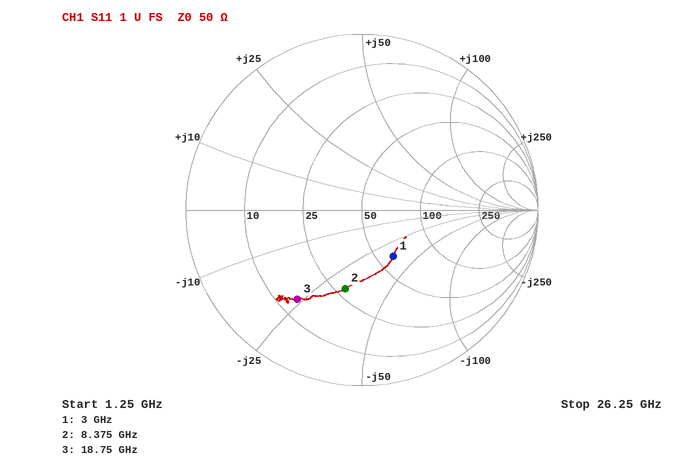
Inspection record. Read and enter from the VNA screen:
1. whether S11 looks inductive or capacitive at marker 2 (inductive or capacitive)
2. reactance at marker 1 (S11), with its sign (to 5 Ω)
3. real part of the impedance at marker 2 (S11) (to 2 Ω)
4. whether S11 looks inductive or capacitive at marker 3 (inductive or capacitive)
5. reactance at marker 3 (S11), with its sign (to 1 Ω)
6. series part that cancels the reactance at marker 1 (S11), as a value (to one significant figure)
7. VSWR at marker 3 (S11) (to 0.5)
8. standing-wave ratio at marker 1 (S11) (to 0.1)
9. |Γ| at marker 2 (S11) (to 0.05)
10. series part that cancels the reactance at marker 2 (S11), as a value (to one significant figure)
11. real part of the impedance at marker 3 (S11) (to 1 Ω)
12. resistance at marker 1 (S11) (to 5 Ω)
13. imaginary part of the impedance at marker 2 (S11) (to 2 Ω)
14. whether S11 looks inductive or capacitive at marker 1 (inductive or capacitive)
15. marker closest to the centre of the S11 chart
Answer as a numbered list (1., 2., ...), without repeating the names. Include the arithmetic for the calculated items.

1. capacitive
2. -35 Ω
3. 28 Ω
4. capacitive
5. -24 Ω
6. L = 35 Ω/(2π × 3 GHz) ≈ 2 nH
7. 4.5
8. 1.9
9. 0.45
10. L = 32 Ω/(2π × 8.375 GHz) ≈ 608 pH, so 600 pH to one significant figure
11. 14 Ω
12. 60 Ω
13. -32 Ω
14. capacitive
15. marker 1
